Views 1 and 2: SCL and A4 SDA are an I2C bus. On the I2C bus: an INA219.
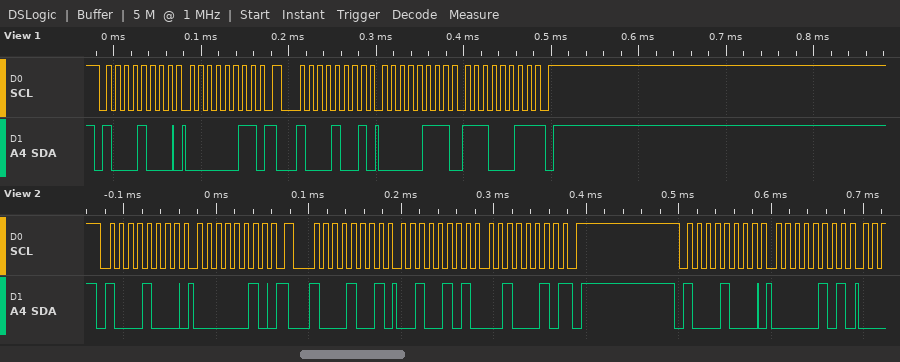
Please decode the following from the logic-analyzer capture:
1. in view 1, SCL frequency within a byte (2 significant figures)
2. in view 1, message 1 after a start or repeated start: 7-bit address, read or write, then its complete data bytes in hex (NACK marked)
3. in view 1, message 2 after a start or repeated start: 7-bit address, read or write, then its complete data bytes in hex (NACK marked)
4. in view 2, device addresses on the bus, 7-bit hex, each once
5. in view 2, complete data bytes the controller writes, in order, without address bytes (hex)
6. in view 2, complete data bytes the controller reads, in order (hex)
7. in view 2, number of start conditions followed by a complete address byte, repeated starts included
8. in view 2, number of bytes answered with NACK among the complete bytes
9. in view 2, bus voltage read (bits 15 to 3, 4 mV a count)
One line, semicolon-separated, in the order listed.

100 kHz; 0x44 write: 03; 0x44 read: 07 E3 NACK; 0x44; 02 05; 25 22; 3; 1; 4.752 V
